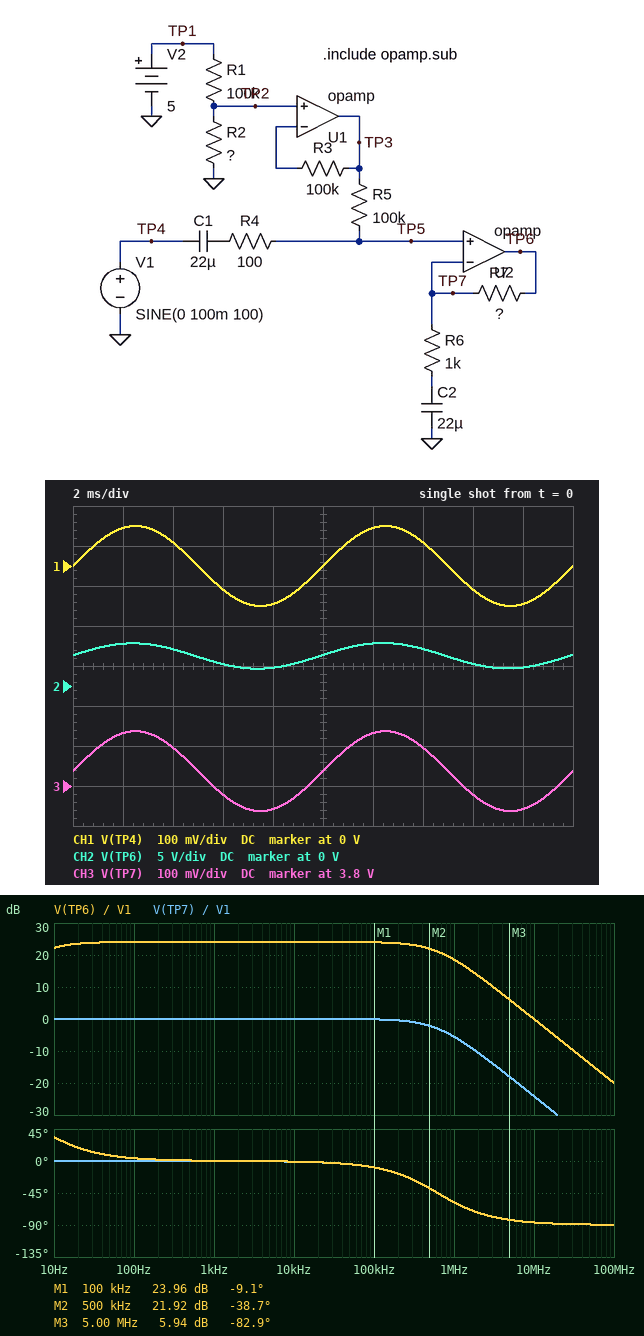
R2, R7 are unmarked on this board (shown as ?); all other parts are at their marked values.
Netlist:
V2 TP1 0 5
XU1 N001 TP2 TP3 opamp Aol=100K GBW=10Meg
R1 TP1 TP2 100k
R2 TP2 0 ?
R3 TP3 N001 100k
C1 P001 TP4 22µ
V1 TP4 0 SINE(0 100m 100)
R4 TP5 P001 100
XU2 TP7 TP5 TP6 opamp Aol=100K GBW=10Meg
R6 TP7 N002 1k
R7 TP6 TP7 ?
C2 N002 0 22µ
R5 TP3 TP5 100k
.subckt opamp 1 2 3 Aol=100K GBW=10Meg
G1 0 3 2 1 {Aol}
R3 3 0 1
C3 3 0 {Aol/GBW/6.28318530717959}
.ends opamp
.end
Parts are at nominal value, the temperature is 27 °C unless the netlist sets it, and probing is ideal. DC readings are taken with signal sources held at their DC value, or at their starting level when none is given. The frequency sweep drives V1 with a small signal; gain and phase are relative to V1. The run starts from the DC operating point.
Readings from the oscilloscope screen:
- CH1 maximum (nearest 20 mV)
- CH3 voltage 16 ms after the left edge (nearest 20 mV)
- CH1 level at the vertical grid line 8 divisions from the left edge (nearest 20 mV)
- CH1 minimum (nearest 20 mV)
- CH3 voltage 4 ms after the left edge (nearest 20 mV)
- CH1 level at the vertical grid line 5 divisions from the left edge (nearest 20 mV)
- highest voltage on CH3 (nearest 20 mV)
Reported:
100 mV
3.78 V
-60 mV
-100 mV
3.90 V
0 V
3.94 V
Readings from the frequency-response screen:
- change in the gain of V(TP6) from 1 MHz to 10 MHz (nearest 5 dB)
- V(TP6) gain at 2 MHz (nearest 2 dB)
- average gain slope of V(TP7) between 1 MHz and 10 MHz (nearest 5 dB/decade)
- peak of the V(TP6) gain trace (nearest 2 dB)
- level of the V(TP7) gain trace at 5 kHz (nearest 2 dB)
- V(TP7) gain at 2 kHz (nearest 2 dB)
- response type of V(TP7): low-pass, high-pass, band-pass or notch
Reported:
-20 dB
14 dB
-20 dB/decade
24 dB
0 dB
0 dB
low-pass
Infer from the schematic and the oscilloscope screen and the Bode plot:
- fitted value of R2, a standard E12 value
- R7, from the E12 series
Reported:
330 kΩ
15 kΩ
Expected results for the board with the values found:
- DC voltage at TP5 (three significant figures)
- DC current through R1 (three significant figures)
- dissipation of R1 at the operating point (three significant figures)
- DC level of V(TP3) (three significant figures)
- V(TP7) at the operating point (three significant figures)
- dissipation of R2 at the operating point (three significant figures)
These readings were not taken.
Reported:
3.84 V
11.6 µA
13.5 µW
3.84 V
3.84 V
44.6 µW
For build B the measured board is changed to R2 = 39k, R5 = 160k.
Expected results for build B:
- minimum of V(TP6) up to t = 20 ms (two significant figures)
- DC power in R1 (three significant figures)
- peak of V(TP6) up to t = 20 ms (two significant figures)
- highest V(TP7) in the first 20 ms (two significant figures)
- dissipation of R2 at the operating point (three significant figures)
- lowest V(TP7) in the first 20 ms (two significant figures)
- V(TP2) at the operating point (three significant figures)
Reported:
-270 mV
129 µW
2.9 V
1.5 V
50.5 µW
1.3 V
1.40 V
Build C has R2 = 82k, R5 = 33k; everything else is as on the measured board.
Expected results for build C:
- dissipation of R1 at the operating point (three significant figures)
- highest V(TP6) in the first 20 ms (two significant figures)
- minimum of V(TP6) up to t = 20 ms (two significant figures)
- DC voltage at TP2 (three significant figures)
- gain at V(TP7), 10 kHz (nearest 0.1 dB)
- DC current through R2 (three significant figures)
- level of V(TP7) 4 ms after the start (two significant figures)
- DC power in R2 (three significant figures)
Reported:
75.5 µW
3.8 V
580 mV
2.25 V
0 dB
27.5 µA
2.3 V
61.9 µW
